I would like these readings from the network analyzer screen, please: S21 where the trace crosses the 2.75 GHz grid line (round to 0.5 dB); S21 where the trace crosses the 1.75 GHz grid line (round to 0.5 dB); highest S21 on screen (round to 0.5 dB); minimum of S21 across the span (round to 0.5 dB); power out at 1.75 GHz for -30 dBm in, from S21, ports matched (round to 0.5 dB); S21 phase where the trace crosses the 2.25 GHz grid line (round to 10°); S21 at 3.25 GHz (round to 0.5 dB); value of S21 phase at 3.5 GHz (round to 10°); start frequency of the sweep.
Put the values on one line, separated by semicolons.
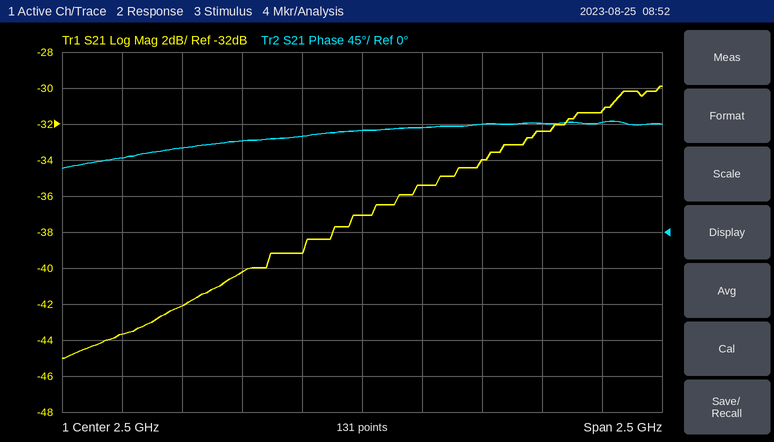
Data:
-35.5 dB; -42.0 dB; -30.0 dB; -45.0 dB; -72.0 dBm; 120°; -32.5 dB; 140°; 1.25 GHz
